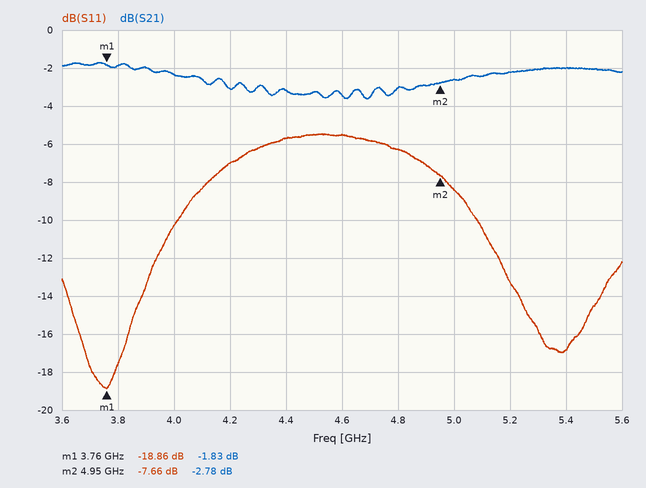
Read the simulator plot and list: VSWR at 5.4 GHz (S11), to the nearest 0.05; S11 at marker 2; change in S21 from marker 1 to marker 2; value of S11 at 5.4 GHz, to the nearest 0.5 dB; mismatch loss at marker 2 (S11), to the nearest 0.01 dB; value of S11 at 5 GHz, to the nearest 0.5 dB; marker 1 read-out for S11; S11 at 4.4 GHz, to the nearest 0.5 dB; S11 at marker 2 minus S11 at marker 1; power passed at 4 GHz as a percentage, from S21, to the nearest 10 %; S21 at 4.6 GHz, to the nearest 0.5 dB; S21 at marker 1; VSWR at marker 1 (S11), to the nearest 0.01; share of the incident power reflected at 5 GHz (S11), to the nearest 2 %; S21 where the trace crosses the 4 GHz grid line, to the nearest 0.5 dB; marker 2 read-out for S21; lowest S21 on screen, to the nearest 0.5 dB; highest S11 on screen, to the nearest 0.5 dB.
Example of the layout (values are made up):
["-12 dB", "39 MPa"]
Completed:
["1.35", "-7.66 dB", "-0.95 dB", "-17.0 dB", "0.82 dB", "-8.5 dB", "-18.86 dB", "-5.5 dB", "11.20 dB", "60 %", "-3.5 dB", "-1.83 dB", "1.26", "14 %", "-2.5 dB", "-2.78 dB", "-3.5 dB", "-5.5 dB"]
